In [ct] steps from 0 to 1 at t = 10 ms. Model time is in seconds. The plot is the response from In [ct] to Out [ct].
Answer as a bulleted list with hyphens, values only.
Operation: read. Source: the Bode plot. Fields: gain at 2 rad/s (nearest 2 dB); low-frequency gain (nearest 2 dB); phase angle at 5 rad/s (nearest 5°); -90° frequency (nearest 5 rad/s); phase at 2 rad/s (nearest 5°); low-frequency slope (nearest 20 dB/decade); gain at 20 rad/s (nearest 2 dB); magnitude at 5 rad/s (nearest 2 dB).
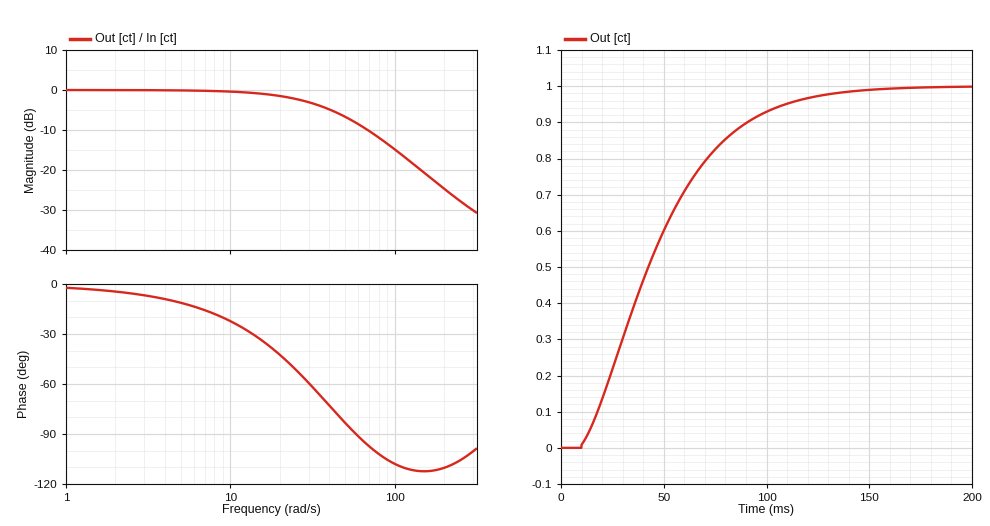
- 0 dB
- 0 dB
- -10°
- 60 rad/s
- -5°
- 0 dB/decade
- -2 dB
- 0 dB
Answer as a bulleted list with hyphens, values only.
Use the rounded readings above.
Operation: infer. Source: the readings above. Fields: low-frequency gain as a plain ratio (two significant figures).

- 1.0
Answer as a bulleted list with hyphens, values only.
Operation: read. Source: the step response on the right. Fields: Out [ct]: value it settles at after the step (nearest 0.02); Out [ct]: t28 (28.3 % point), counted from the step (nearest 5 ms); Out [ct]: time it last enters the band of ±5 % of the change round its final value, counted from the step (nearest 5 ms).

- 1.00
- 20 ms
- 100 ms
